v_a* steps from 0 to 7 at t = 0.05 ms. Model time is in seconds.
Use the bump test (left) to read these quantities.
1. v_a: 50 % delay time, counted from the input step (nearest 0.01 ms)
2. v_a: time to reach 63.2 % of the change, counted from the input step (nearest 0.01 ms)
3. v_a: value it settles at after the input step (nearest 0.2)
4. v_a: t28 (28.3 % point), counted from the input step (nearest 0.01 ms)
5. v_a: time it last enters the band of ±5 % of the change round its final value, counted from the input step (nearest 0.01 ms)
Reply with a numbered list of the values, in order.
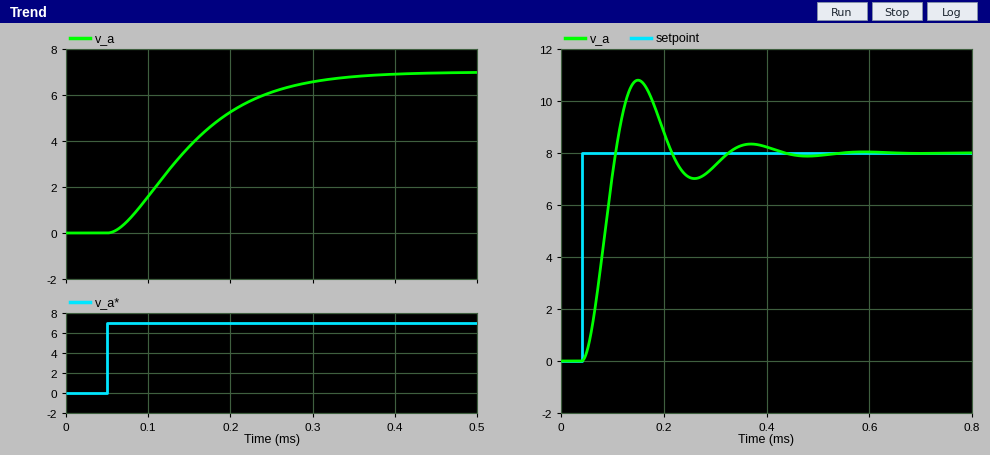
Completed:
1. 0.09 ms
2. 0.12 ms
3. 7.0
4. 0.06 ms
5. 0.26 ms
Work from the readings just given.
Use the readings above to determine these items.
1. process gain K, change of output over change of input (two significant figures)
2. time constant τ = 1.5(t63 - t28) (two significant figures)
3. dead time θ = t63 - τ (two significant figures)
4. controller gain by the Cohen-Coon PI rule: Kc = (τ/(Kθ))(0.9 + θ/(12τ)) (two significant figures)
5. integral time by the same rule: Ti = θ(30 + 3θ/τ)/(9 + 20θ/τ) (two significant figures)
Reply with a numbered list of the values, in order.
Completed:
1. 1.0
2. 0.090 ms
3. 0.030 ms
4. 2.8
5. 0.059 ms
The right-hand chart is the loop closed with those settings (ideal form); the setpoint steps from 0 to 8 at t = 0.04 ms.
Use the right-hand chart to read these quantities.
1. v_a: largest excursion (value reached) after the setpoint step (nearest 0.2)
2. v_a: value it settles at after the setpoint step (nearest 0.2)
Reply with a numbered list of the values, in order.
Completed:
1. 10.8
2. 8.0
